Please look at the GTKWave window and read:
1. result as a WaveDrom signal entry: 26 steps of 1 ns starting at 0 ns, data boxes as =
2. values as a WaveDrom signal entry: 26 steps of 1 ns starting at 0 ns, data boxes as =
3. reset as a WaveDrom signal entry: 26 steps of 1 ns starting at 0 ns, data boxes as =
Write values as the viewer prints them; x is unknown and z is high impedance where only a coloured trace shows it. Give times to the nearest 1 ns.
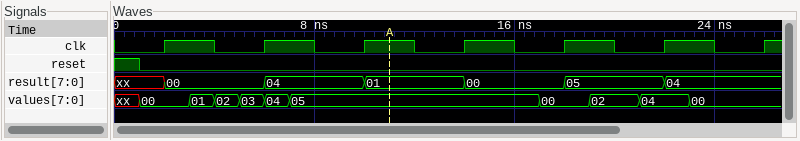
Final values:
{name: 'result', wave: 'x.=...=...=...=...=...=...', data: '00 04 01 00 05 04'}
{name: 'values', wave: 'x=.=====.........=.=.=.=..', data: '00 01 02 03 04 05 00 02 04 00'}
{name: 'reset', wave: '10........................'}
